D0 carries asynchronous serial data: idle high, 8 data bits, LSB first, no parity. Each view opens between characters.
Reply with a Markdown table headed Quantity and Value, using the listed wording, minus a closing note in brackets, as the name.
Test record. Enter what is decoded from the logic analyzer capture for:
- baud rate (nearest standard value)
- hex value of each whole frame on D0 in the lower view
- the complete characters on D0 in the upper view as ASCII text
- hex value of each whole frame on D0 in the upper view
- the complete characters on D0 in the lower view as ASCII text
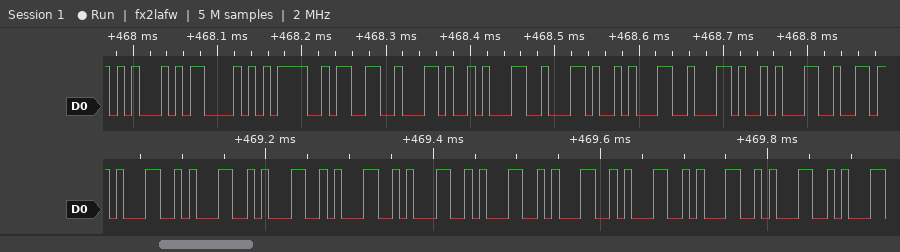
| Quantity | Value |
|---|---|
| baud rate | 115200 baud |
| hex value of each whole frame on D0 in the lower view | 31, 31, 31, 31, 31, 31, 31, 31, 31, 31 |
| the complete characters on D0 in the upper view as ASCII text | "EC=3,1,1,1" |
| hex value of each whole frame on D0 in the upper view | 45, 43, 3D, 33, 2C, 31, 2C, 31, 2C, 31 |
| the complete characters on D0 in the lower view as ASCII text | "1111111111" |
